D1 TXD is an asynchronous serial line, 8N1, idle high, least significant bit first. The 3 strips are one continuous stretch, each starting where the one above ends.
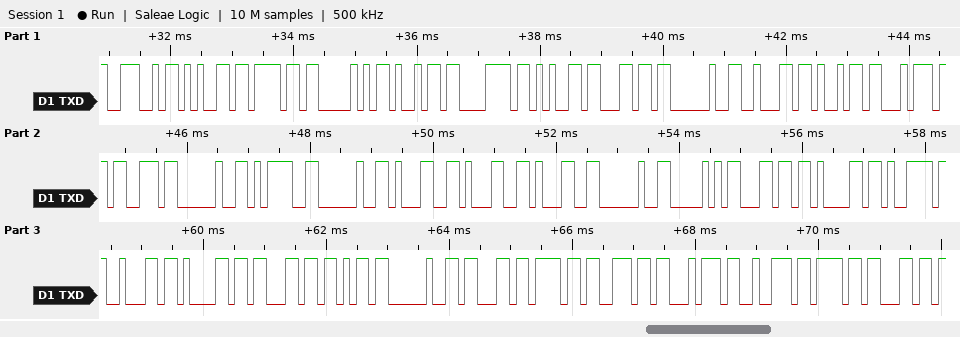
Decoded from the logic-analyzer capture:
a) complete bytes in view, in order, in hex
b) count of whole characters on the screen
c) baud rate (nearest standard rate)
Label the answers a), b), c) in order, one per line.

a) 4E 65 6F 50 69 78 65 6C 20 62 69 74 73 20 3D 20 31 31 31 20 50 6C 61 79 62 61 63 6B 20 63 6F 6E 74 72 6F 6C
b) 36
c) 9600 baud
